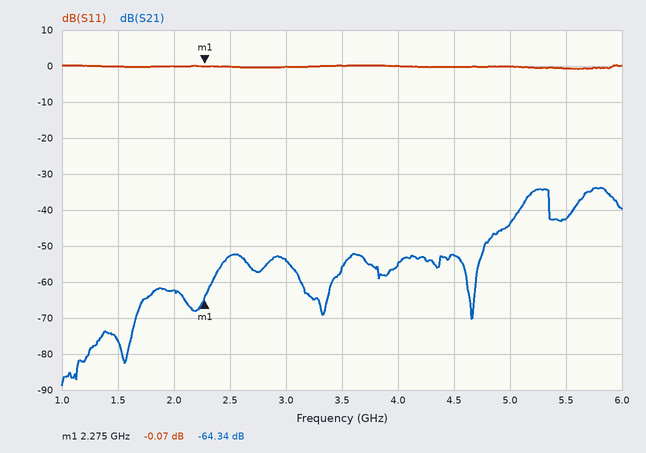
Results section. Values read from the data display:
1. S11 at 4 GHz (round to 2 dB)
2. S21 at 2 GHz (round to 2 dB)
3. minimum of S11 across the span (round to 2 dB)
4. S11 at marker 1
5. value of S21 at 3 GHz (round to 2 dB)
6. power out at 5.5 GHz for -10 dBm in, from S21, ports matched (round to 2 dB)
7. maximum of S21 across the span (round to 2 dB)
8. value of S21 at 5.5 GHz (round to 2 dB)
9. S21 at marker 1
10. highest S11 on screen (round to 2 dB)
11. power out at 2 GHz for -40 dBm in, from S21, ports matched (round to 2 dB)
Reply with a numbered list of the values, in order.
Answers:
1. 0 dB
2. -62 dB
3. 0 dB
4. -0.07 dB
5. -54 dB
6. -52 dBm
7. -34 dB
8. -42 dB
9. -64.34 dB
10. 0 dB
11. -102 dBm
